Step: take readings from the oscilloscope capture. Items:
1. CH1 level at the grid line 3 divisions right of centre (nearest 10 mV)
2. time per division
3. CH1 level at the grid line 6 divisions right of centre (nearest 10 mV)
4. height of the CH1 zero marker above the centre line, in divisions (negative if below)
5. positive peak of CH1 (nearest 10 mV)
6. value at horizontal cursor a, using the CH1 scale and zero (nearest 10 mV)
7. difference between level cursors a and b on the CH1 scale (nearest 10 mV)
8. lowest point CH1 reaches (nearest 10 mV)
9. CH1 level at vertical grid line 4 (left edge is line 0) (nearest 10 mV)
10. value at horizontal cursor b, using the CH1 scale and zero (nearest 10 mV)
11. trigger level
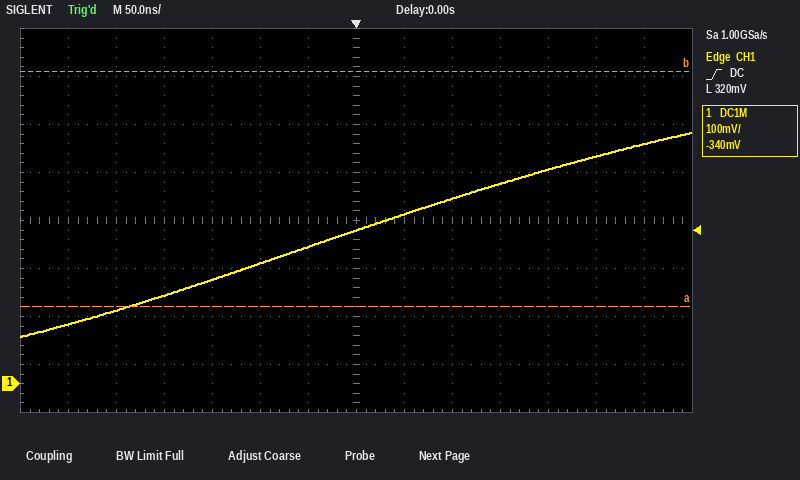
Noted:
420 mV
50 ns
500 mV
-3.4 div
520 mV
160 mV
490 mV
100 mV
220 mV
650 mV
320 mV
